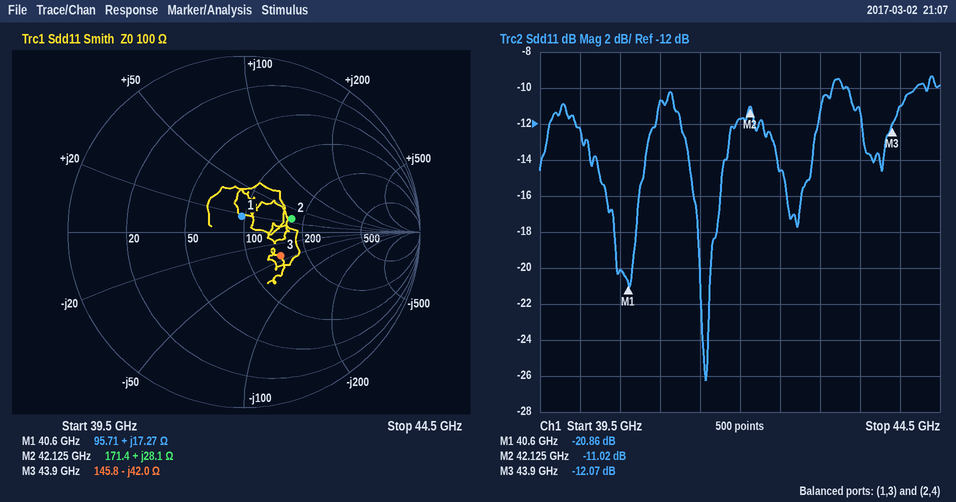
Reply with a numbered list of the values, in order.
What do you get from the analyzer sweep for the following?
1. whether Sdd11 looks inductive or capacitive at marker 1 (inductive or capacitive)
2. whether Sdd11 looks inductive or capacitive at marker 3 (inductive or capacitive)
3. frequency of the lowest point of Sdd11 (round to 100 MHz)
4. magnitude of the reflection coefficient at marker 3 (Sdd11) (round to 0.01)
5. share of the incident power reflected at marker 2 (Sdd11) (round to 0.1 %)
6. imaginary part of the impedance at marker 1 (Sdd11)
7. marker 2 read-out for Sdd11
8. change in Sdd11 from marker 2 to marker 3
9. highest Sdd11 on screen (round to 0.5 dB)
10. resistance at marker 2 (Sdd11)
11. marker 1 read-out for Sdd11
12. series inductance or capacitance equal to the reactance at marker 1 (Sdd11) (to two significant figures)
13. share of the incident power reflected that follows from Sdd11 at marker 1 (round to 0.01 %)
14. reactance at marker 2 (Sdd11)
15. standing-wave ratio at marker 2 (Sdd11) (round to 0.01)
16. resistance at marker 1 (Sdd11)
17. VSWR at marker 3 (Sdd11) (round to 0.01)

1. inductive
2. capacitive
3. 41.6 GHz
4. 0.25
5. 7.9 %
6. +17.27 Ω
7. -11.02 dB
8. -1.05 dB
9. -9.5 dB
10. 171.4 Ω
11. -20.86 dB
12. 68 pH
13. 0.82 %
14. +28.1 Ω
15. 1.78
16. 95.71 Ω
17. 1.66
